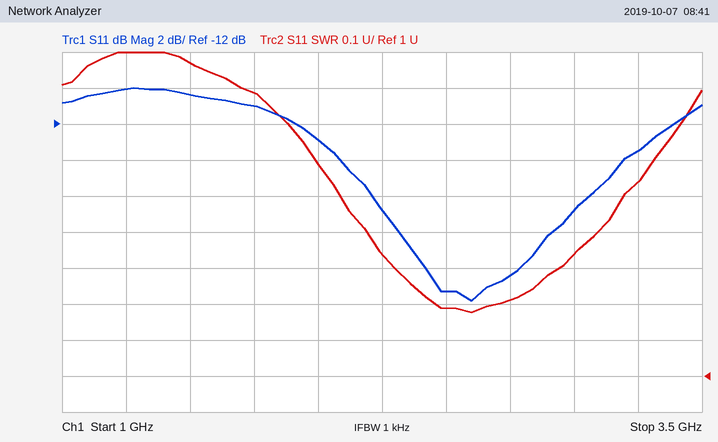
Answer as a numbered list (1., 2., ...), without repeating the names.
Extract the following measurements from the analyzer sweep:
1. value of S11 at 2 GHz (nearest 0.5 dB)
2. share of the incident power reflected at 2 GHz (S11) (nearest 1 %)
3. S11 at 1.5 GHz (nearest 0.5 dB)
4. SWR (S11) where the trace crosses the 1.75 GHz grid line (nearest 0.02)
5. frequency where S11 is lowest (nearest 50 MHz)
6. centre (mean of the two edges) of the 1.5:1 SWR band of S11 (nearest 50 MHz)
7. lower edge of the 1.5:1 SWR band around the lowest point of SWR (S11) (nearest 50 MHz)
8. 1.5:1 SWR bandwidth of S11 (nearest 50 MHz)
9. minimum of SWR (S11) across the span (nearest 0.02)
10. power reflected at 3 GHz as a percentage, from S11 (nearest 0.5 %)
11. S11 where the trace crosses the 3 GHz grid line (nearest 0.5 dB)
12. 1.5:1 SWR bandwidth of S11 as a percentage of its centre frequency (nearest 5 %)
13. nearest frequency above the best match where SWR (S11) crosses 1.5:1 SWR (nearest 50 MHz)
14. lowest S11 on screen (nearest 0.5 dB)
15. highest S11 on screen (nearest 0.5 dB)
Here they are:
1. -13.0 dB
2. 5 %
3. -10.5 dB
4. 1.78
5. 2.60 GHz
6. 2.65 GHz
7. 2.10 GHz
8. 1.10 GHz
9. 1.18
10. 2.0 %
11. -17.0 dB
12. 40 %
13. 3.20 GHz
14. -22.0 dB
15. -10.0 dB
